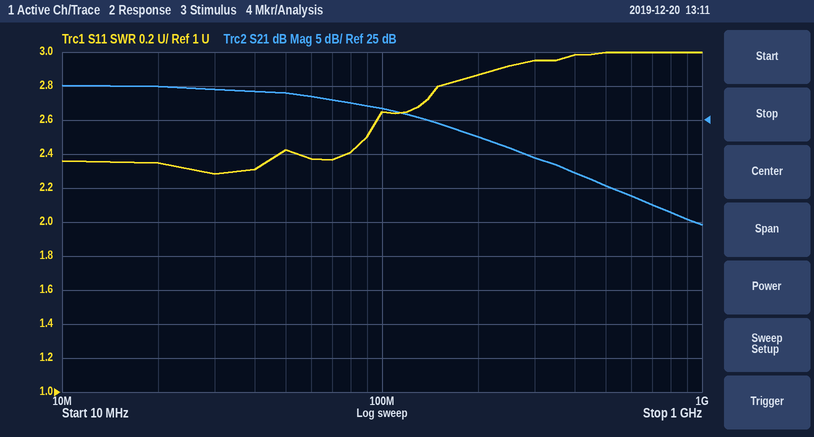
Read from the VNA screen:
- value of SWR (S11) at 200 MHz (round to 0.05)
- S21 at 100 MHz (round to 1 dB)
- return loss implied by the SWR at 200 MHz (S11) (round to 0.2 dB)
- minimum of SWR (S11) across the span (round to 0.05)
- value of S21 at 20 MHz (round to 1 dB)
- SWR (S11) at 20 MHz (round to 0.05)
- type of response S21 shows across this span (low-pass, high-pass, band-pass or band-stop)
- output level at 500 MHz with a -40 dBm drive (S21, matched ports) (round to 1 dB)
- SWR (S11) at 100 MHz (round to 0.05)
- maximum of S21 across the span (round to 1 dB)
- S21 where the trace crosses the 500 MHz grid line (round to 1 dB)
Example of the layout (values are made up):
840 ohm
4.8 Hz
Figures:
2.85
27 dB
6.4 dB
2.30
30 dB
2.35
low-pass
-25 dBm
2.65
30 dB
15 dB
